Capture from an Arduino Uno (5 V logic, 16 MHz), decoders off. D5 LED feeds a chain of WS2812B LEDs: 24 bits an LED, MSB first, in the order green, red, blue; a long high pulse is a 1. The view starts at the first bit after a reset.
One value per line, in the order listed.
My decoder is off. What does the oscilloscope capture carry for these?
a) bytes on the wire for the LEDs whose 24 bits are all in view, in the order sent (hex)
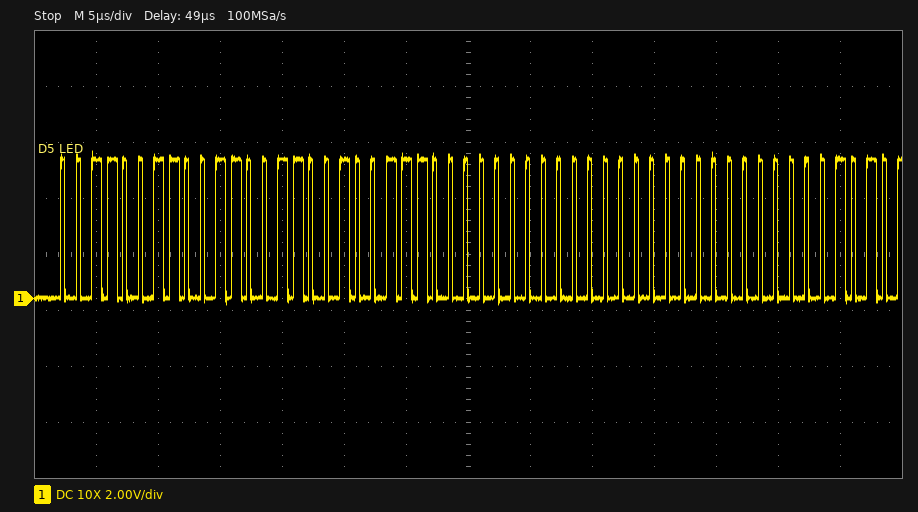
33 33 27 00 00 00
